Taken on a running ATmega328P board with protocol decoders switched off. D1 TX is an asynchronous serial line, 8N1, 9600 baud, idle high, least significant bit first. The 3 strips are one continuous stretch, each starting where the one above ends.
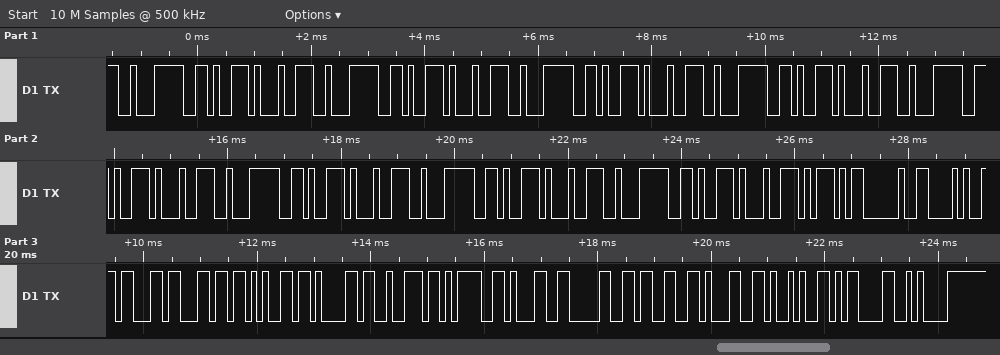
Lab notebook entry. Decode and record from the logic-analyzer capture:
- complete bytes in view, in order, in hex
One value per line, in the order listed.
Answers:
E2 96 91 E2 96 91 E2 96 91 E2 96 91 E2 96 91 E2 96 91 E2 96 91 E2 96 91 5D 20 28 63 6C 65 61 72 3D 31 30 33 31 29 0D 0A
